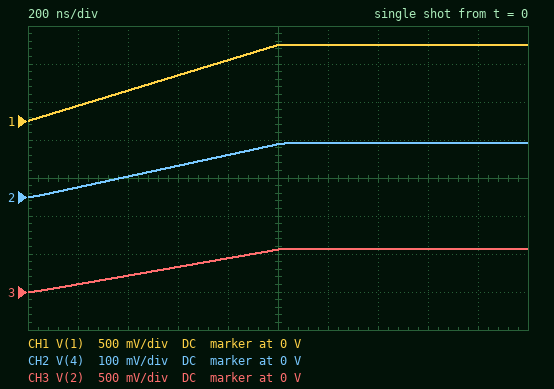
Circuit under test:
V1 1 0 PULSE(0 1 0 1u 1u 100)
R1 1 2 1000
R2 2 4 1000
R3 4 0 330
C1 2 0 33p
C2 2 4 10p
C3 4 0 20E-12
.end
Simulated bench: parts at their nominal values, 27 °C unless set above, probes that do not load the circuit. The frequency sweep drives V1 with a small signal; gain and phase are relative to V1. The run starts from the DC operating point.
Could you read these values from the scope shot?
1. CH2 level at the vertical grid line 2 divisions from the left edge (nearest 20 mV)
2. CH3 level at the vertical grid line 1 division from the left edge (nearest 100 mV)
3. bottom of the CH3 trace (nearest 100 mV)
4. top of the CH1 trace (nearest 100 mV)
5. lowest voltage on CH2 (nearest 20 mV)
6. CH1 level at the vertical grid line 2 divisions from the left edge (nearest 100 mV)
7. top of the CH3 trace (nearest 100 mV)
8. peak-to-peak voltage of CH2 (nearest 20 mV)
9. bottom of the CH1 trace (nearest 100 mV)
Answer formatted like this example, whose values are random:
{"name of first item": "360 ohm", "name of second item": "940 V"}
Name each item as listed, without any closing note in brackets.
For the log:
{"CH2 level at the vertical grid line 2 divisions from the left edge": "60 mV", "CH3 level at the vertical grid line 1 division from the left edge": "100 mV", "bottom of the CH3 trace": "0 V", "top of the CH1 trace": "1.0 V", "lowest voltage on CH2": "0 V", "CH1 level at the vertical grid line 2 divisions from the left edge": "400 mV", "top of the CH3 trace": "600 mV", "peak-to-peak voltage of CH2": "140 mV", "bottom of the CH1 trace": "0 V"}
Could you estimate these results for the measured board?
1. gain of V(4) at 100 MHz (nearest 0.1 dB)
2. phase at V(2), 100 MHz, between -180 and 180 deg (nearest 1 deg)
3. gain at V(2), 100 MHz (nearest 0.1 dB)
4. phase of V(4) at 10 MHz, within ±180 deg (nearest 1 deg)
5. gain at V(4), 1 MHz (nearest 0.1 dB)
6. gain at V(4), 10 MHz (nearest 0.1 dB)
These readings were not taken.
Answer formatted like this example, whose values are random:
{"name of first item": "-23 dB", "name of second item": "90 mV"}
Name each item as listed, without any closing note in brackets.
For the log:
{"gain of V(4) at 100 MHz": "-37.6 dB", "phase at V(2), 100 MHz, between -180 and 180 deg": "-86 deg", "gain at V(2), 100 MHz": "-28.0 dB", "phase of V(4) at 10 MHz, within ±180 deg": "-48 deg", "gain at V(4), 1 MHz": "-17.1 dB", "gain at V(4), 10 MHz": "-21.2 dB"}
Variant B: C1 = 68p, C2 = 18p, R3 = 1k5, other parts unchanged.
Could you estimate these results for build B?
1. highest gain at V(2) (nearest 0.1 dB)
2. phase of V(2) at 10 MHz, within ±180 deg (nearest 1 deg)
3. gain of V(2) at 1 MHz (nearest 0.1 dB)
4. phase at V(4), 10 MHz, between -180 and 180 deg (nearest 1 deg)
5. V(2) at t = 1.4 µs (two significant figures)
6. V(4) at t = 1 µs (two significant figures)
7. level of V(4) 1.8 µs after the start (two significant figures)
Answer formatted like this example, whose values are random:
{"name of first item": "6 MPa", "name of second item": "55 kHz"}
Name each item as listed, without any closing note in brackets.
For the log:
{"highest gain at V(2)": "-2.9 dB", "phase of V(2) at 10 MHz, within ±180 deg": "-74 deg", "gain of V(2) at 1 MHz": "-3.4 dB", "phase at V(4), 10 MHz, between -180 and 180 deg": "-80 deg", "V(2) at t = 1.4 µs": "710 mV", "V(4) at t = 1 µs": "400 mV", "level of V(4) 1.8 µs after the start": "430 mV"}
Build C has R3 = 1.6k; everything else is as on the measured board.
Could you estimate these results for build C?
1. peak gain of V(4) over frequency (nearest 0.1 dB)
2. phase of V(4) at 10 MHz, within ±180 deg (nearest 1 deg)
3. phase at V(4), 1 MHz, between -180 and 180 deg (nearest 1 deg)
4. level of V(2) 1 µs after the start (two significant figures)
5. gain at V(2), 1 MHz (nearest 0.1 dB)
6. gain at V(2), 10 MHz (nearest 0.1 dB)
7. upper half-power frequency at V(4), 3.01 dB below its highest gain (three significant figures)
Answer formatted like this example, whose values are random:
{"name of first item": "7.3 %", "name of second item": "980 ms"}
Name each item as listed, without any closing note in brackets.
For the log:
{"peak gain of V(4) over frequency": "-7.0 dB", "phase of V(4) at 10 MHz, within ±180 deg": "-77 deg", "phase at V(4), 1 MHz, between -180 and 180 deg": "-14 deg", "level of V(2) 1 µs after the start": "700 mV", "gain at V(2), 1 MHz": "-3.0 dB", "gain at V(2), 10 MHz": "-9.4 dB", "upper half-power frequency at V(4), 3.01 dB below its highest gain": "4.35 MHz"}
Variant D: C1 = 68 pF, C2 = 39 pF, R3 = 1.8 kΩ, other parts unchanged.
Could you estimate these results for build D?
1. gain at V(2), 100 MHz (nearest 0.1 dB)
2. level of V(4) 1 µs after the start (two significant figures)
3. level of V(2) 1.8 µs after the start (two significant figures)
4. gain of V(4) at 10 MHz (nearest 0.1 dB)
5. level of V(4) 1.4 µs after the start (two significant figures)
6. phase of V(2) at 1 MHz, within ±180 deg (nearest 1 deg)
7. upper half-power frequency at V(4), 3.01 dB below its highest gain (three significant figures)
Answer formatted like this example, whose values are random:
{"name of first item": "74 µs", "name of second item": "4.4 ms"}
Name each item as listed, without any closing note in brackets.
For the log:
{"gain at V(2), 100 MHz": "-34.2 dB", "level of V(4) 1 µs after the start": "450 mV", "level of V(2) 1.8 µs after the start": "740 mV", "gain of V(4) at 10 MHz": "-18.1 dB", "level of V(4) 1.4 µs after the start": "470 mV", "phase of V(2) at 1 MHz, within ±180 deg": "-21 deg", "upper half-power frequency at V(4), 3.01 dB below its highest gain": "2.70 MHz"}
